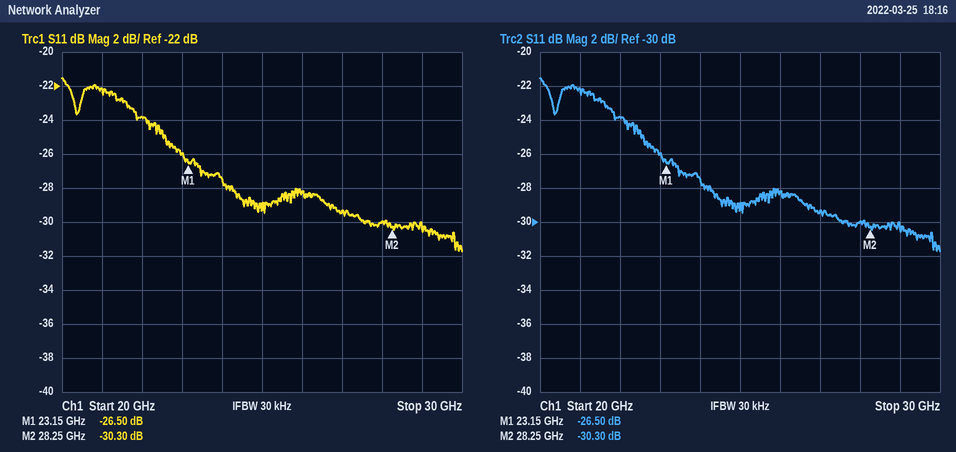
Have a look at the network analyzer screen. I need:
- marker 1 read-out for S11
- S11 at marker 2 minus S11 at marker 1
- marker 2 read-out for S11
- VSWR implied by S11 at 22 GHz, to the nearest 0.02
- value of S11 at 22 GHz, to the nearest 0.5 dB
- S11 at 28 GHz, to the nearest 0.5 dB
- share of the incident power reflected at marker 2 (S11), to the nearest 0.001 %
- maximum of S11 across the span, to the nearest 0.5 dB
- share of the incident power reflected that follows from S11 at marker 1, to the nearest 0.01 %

-26.50 dB
-3.80 dB
-30.30 dB
1.14
-24.0 dB
-30.0 dB
0.093 %
-21.5 dB
0.22 %
